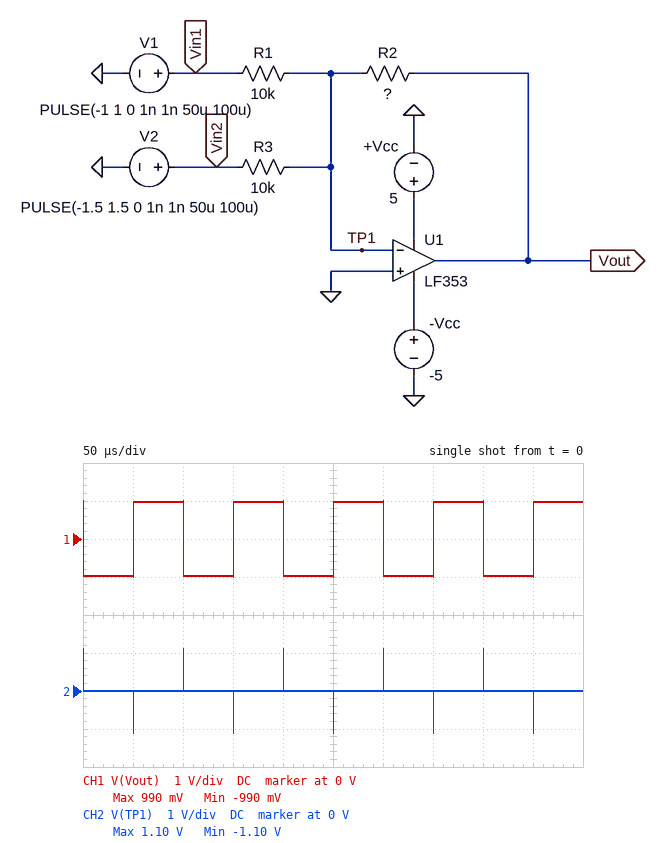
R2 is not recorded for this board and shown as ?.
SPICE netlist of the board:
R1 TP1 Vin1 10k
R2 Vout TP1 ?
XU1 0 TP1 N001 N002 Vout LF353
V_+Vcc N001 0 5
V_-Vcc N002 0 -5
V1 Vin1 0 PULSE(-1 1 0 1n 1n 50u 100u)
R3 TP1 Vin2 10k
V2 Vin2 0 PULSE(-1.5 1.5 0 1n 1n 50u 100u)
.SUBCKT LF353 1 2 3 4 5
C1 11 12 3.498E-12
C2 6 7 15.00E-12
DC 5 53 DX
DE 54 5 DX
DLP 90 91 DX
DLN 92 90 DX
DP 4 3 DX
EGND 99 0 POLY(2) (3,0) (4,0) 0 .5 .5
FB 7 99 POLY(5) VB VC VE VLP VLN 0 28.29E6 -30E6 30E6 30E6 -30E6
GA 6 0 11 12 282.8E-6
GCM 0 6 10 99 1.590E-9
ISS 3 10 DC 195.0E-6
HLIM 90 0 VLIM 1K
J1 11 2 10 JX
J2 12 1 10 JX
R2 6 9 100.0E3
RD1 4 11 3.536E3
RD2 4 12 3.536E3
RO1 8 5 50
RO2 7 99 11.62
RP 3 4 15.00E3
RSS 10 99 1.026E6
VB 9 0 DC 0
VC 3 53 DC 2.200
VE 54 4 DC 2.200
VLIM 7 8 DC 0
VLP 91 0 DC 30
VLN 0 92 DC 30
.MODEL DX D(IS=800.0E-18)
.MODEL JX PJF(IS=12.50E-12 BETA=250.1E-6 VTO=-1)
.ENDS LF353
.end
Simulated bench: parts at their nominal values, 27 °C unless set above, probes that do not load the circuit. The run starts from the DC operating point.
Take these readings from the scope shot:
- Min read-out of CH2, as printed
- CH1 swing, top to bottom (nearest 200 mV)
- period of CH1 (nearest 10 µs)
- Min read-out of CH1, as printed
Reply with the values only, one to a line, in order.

-1.10 V
2.0 V
100 µs
-990 mV
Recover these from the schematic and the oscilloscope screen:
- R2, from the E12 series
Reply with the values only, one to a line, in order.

3.9 kΩ
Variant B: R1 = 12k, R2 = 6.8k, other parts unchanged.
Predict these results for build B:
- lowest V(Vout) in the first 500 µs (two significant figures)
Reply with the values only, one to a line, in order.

-1.6 V
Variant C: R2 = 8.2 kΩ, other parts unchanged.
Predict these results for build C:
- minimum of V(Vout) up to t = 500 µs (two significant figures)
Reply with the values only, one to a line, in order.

-2.1 V
